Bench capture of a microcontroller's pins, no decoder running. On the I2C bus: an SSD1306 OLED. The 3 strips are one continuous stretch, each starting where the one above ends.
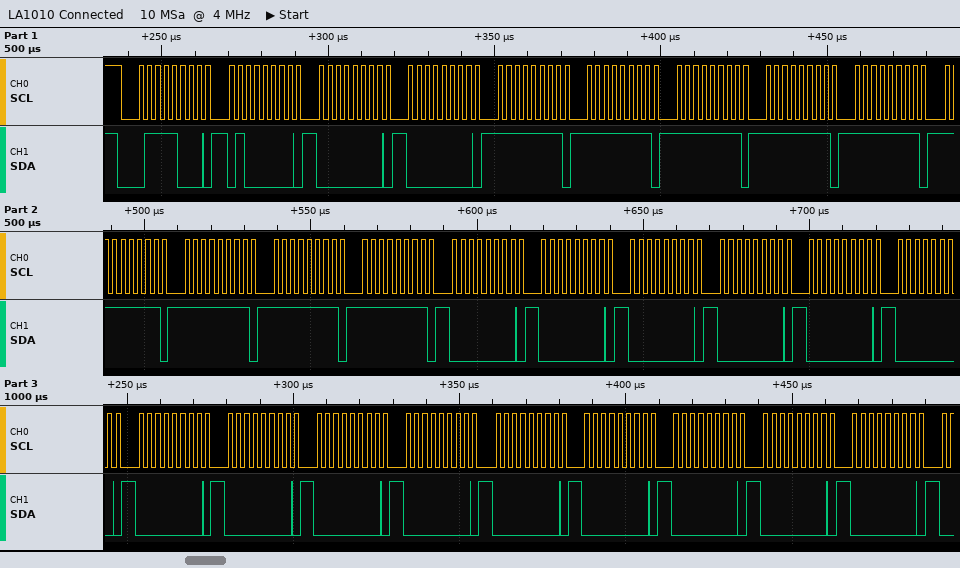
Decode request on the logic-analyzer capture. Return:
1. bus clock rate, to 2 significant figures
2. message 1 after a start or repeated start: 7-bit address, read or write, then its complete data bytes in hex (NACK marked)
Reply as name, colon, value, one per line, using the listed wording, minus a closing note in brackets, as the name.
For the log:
bus clock rate, to 2 significant figures: 400 kHz
message 1 after a start or repeated start: 7-bit address, read or write, then its complete data bytes in hex: 0x3C write: 40 00 00 FF FF FF FF FF FF FF FF FF 00 00 00 00 00 00 00 00 00 00 00 00 00 00 00
